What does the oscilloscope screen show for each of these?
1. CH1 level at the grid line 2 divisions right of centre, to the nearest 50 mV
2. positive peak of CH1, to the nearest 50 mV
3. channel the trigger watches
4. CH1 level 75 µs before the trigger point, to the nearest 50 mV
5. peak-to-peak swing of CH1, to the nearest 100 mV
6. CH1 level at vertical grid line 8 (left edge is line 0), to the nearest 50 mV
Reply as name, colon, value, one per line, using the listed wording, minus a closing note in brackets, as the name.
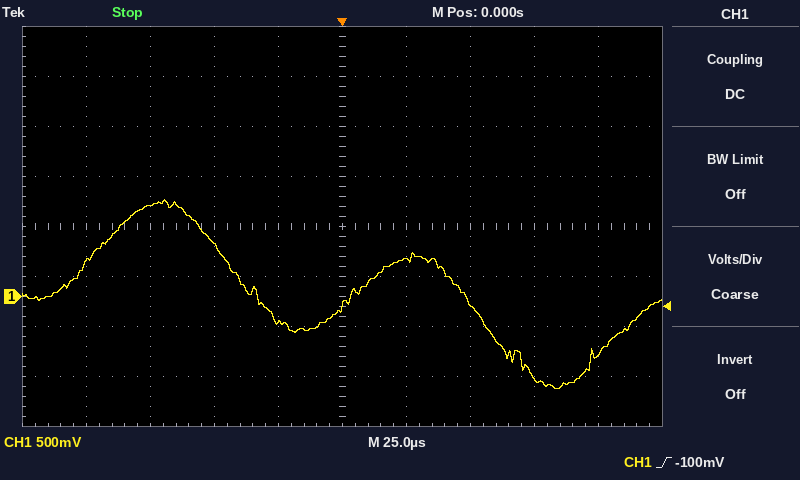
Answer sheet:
CH1 level at the grid line 2 divisions right of centre, to the nearest 50 mV: -50 mV
positive peak of CH1, to the nearest 50 mV: 950 mV
channel the trigger watches: CH1
CH1 level 75 µs before the trigger point, to the nearest 50 mV: 900 mV
peak-to-peak swing of CH1, to the nearest 100 mV: 1.90 V
CH1 level at vertical grid line 8 (left edge is line 0), to the nearest 50 mV: -800 mV
